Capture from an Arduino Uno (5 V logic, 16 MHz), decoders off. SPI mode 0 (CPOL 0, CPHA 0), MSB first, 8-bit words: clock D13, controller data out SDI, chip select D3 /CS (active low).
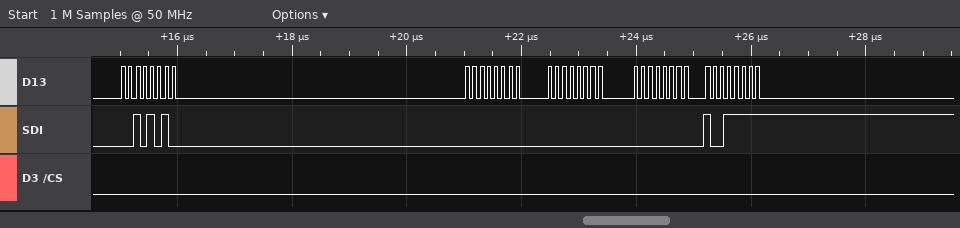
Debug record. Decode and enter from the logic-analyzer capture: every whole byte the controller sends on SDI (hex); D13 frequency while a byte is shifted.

2A 00 00 00 9F
8 MHz
